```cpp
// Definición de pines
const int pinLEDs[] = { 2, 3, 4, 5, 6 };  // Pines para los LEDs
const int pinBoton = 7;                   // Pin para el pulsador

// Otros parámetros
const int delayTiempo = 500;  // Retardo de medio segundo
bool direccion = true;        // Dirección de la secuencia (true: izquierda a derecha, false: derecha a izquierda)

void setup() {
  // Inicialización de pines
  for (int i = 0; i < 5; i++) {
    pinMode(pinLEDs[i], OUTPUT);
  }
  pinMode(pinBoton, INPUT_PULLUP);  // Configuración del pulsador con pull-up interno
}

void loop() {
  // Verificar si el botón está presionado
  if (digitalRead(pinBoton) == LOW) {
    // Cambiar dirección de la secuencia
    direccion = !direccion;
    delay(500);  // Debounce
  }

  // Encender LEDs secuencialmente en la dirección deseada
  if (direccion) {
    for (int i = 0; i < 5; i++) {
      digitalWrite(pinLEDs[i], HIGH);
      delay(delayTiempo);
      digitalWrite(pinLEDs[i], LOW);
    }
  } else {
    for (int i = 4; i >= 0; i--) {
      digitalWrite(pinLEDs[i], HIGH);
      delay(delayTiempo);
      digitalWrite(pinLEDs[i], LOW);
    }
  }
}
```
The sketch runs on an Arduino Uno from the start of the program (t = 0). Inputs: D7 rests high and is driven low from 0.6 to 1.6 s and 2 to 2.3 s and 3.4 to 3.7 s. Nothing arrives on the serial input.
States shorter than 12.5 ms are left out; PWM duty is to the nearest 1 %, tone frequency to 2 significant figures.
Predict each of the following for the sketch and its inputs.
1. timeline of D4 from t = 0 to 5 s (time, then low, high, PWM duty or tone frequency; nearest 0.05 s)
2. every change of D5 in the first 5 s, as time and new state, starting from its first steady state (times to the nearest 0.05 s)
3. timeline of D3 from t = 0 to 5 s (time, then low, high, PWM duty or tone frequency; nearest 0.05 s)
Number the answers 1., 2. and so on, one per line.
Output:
1. 0 s low; 1 s high; 1.5 s low; 3.5 s high; 4 s low
2. 0 s low; 1.5 s high; 2 s low; 4 s high; 4.5 s low
3. 0 s low; 0.5 s high; 1 s low; 3 s high; 3.5 s low
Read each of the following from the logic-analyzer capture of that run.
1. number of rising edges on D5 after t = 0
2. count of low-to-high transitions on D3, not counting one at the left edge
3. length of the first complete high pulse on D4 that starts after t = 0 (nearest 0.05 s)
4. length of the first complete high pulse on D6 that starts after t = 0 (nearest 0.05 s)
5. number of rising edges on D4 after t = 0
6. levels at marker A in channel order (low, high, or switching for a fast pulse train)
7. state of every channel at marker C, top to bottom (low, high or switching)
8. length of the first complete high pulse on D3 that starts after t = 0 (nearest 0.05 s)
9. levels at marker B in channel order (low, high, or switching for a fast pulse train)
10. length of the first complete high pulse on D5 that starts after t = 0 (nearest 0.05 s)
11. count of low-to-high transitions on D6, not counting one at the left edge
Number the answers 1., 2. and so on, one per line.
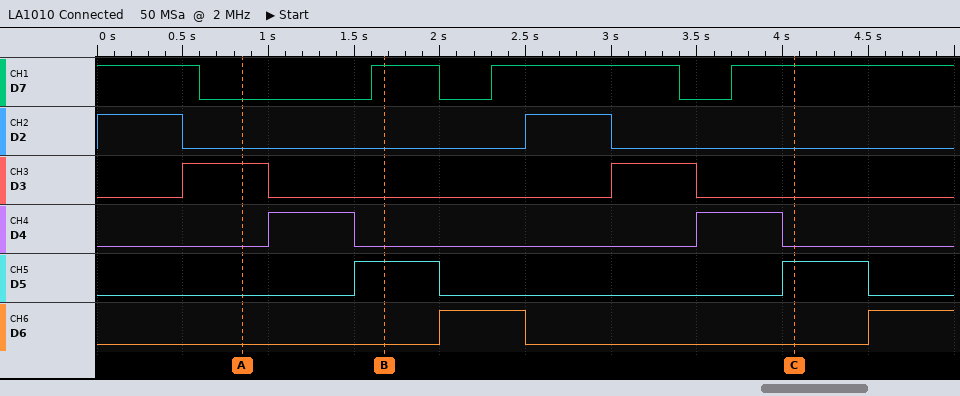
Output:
1. 2
2. 2
3. 0.50 s
4. 0.50 s
5. 2
6. D7 low, D2 low, D3 high, D4 low, D5 low, D6 low
7. D7 high, D2 low, D3 low, D4 low, D5 high, D6 low
8. 0.50 s
9. D7 high, D2 low, D3 low, D4 low, D5 high, D6 low
10. 0.50 s
11. 2
